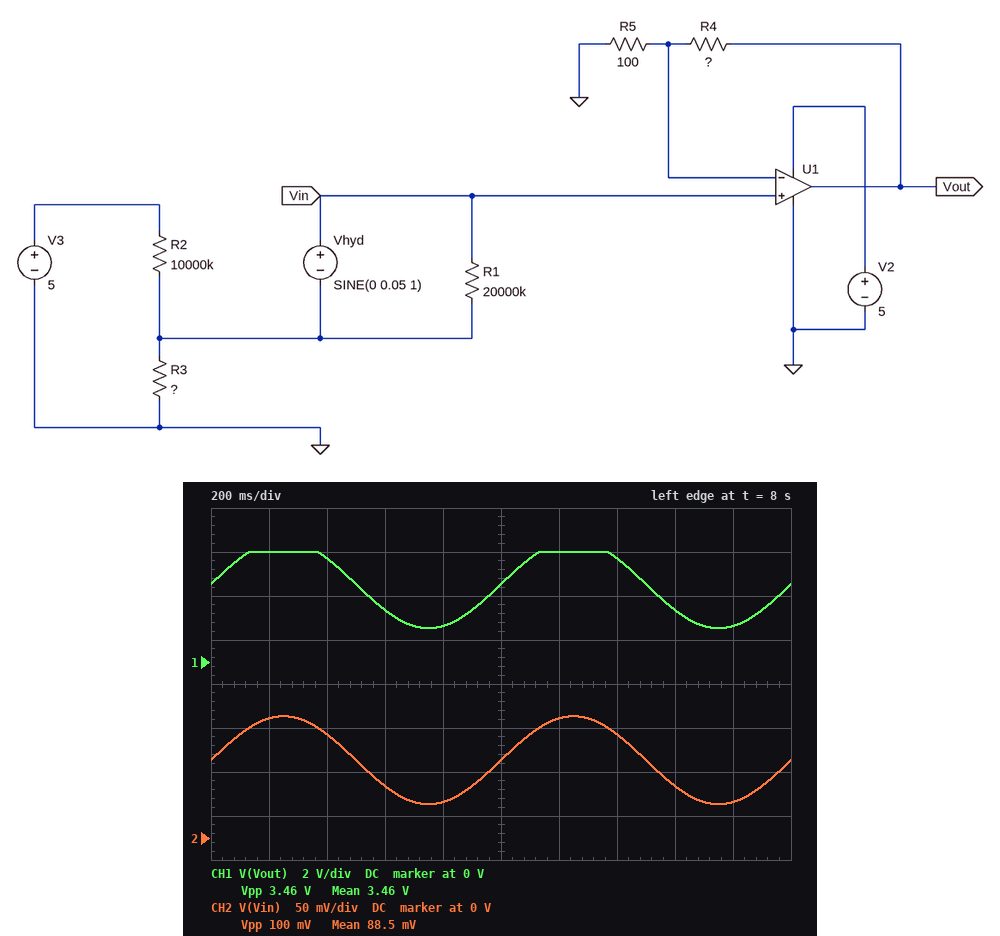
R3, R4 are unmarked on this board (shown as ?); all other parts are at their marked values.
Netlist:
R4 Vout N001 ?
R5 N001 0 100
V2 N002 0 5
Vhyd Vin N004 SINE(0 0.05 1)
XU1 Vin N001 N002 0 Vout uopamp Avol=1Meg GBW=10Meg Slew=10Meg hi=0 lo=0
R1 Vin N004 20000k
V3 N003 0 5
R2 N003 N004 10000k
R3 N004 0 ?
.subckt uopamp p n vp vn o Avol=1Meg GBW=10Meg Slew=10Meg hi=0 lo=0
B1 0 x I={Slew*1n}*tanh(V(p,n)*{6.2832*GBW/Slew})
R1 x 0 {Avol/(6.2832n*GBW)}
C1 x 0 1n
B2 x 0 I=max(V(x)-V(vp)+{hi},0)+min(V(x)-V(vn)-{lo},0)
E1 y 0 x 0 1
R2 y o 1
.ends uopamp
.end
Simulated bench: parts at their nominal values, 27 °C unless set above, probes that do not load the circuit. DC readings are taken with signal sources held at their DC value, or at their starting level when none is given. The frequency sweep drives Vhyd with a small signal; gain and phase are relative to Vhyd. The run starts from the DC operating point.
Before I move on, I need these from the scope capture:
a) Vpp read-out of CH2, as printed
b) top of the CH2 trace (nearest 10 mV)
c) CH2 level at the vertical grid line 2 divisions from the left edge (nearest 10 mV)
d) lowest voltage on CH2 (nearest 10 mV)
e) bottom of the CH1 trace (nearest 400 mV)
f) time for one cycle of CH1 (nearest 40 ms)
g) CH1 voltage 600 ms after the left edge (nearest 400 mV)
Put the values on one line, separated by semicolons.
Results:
100 mV; 140 mV; 120 mV; 40 mV; 1.6 V; 1.00 s; 2.4 V
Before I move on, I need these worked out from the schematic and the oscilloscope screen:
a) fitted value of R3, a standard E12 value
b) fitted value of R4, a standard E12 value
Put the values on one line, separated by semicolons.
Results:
180 kΩ; 3.9 kΩ
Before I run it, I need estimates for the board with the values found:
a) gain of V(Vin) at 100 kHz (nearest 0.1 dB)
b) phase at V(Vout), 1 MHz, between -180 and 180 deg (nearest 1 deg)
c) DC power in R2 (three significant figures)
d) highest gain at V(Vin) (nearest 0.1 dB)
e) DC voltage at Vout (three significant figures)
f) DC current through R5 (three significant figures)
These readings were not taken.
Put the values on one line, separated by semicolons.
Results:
0 dB; -76 deg; 2.41 µW; 0 dB; 3.54 V; 884 µA
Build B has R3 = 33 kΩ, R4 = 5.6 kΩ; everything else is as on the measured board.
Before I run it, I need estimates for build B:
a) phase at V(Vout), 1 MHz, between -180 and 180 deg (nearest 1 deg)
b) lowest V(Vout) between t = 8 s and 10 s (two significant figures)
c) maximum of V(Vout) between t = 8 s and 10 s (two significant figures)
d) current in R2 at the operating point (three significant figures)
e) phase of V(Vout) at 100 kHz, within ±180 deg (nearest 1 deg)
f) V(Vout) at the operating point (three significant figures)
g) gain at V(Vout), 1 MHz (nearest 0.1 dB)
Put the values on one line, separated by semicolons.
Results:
-80 deg; -2.1 mV; 3.8 V; 498 nA; -30 deg; 937 mV; 19.9 dB
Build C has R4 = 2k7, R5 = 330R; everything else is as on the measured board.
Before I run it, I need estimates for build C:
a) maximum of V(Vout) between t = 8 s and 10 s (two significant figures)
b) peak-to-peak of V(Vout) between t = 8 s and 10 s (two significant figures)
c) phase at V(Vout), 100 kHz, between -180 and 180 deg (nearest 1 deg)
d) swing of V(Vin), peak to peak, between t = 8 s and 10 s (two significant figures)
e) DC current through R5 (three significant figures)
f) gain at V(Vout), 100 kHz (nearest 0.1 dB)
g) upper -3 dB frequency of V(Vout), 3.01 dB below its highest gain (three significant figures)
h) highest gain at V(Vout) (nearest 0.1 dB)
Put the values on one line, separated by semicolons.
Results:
1.3 V; 920 mV; -5 deg; 100 mV; 268 µA; 19.2 dB; 1.09 MHz; 19.3 dB
